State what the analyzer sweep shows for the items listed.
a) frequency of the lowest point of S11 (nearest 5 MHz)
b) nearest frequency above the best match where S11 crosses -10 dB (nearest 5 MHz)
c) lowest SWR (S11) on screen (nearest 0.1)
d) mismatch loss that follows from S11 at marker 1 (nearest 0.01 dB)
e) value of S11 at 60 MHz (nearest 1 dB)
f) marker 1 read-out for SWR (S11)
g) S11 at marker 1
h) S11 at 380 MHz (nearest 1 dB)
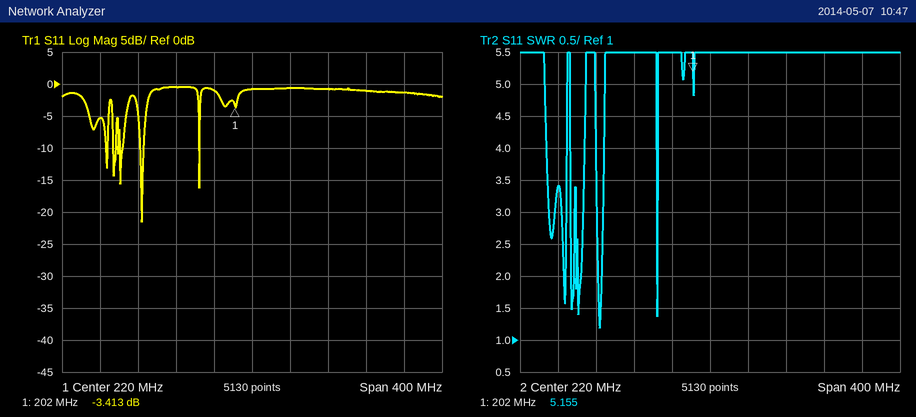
105 MHz
105 MHz
1.2
2.64 dB
-5 dB
5.155
-3.413 dB
-1 dB
